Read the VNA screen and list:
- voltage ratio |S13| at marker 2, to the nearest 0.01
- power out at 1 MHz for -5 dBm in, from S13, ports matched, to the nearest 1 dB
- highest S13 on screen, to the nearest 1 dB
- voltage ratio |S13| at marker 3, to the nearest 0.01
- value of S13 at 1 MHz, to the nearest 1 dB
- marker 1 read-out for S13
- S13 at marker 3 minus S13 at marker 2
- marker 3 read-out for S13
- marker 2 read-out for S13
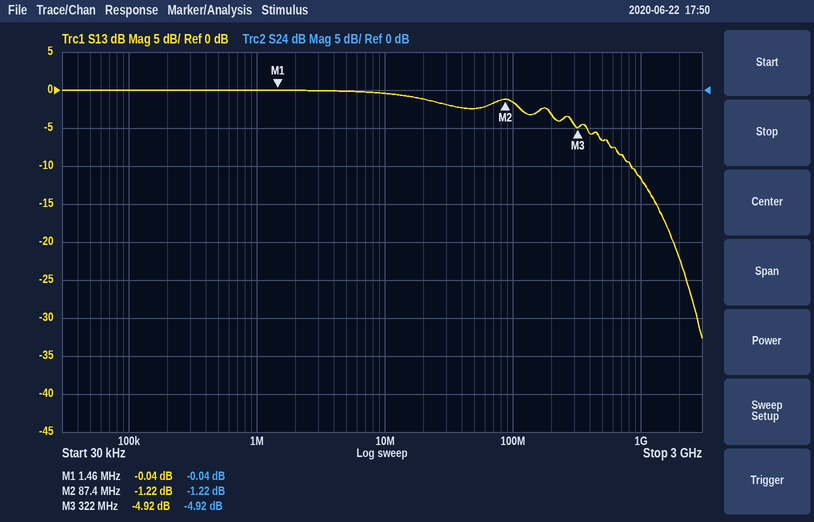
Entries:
0.87
-5 dBm
0 dB
0.57
0 dB
-0.04 dB
-3.70 dB
-4.92 dB
-1.22 dB
